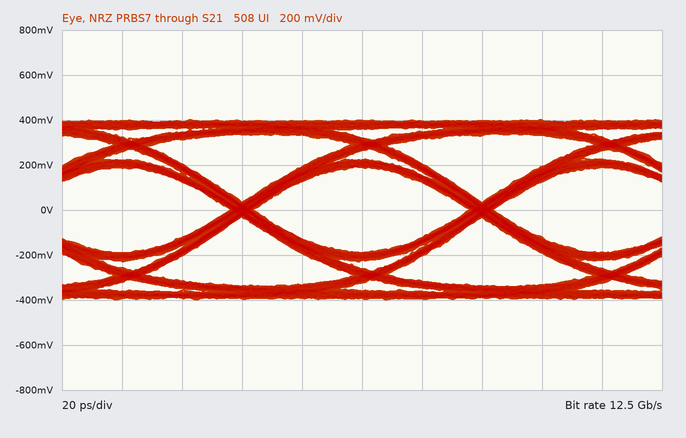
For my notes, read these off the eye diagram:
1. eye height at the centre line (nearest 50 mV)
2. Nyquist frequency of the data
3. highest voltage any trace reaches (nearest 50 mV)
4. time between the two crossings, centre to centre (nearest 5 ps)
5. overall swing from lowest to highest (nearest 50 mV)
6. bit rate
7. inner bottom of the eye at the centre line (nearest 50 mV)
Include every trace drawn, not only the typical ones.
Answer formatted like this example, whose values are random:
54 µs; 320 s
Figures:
400 mV; 6.25 GHz; 400 mV; 80 ps; 800 mV; 12.5 Gb/s; -200 mV
